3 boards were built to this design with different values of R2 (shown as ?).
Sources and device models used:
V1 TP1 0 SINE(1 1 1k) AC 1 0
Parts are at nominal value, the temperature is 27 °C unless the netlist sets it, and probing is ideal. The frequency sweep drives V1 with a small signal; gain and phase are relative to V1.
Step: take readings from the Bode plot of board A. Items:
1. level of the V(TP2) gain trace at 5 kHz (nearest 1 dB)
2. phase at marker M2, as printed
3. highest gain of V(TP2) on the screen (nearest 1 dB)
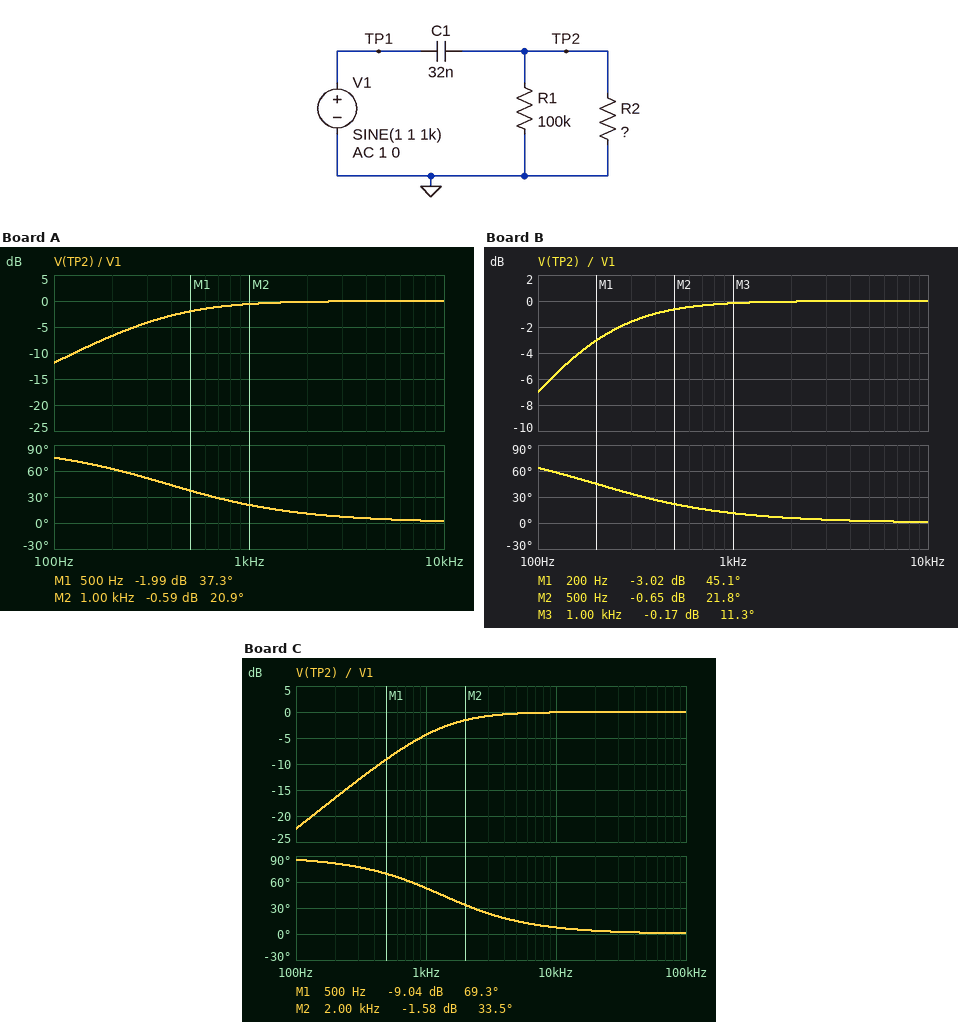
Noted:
0 dB
20.9 deg
0 dB
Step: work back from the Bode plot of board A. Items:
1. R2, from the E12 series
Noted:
15 kΩ
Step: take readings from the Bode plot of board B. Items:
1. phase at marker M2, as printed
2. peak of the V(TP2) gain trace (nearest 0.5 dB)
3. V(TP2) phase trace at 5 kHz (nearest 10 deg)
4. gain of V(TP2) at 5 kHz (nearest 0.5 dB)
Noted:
21.8 deg
0 dB
0 deg
0 dB
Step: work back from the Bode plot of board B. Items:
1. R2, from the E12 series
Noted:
33 kΩ
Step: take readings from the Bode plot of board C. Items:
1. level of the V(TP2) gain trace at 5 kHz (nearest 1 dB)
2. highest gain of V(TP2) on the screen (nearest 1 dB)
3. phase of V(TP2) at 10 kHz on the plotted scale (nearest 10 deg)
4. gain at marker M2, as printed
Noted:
0 dB
0 dB
10 deg
-1.58 dB
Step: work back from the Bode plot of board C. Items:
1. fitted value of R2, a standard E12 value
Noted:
3.9 kΩ
